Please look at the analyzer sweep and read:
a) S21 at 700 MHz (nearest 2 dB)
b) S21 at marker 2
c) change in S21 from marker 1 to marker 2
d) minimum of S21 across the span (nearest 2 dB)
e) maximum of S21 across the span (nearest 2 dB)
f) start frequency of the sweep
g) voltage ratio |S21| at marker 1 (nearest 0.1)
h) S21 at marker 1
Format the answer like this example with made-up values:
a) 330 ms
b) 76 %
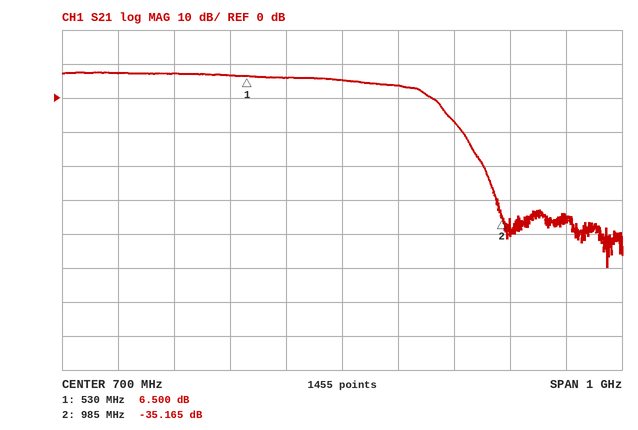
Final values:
a) 6 dB
b) -35.165 dB
c) -41.665 dB
d) -50 dB
e) 8 dB
f) 200 MHz
g) 2.1
h) 6.500 dB
